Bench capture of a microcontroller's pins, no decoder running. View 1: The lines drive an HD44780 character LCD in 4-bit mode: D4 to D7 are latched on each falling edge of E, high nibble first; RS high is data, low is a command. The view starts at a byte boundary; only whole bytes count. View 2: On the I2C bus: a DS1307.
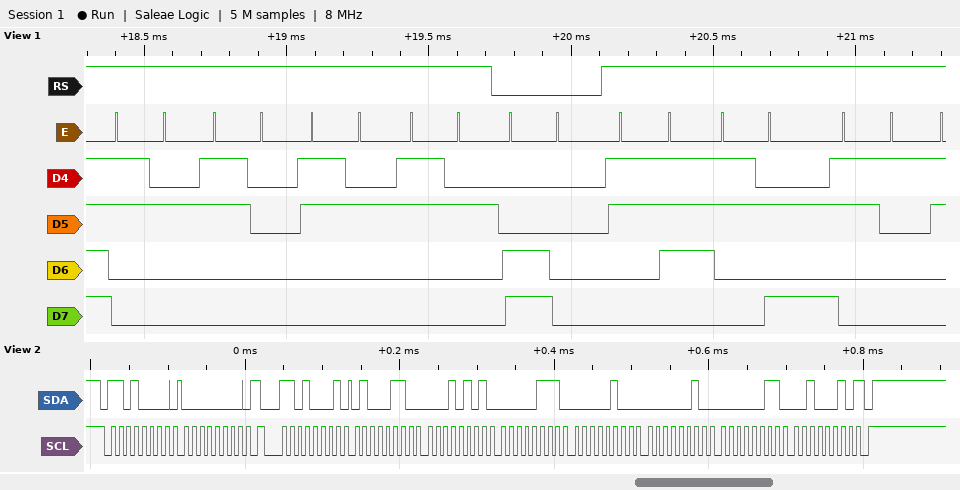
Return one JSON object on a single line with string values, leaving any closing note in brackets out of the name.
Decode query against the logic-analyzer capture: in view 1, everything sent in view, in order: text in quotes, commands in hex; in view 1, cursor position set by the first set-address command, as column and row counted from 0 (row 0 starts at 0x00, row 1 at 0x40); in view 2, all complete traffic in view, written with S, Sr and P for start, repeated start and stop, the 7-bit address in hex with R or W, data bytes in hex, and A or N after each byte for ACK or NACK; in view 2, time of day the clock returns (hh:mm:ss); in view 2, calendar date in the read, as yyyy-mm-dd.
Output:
{"in view 1, everything sent in view, in order: text in quotes, commands in hex": "\"2022\" 0xC0 \"7:1\"", "in view 1, cursor position set by the first set-address command, as column and row counted from 0": "column 0, row 1", "in view 2, all complete traffic in view, written with S, Sr and P for start, repeated start and stop, the 7-bit address in hex with R or W, data bytes in hex, and A or N after each byte for ACK or NACK": "S 68W A 00 A Sr 68R A 46 A 15 A 07 A 04 A 02 A 03 A 22 N P", "in view 2, time of day the clock returns": "07:15:46", "in view 2, calendar date in the read, as yyyy-mm-dd": "2022-03-02"}
